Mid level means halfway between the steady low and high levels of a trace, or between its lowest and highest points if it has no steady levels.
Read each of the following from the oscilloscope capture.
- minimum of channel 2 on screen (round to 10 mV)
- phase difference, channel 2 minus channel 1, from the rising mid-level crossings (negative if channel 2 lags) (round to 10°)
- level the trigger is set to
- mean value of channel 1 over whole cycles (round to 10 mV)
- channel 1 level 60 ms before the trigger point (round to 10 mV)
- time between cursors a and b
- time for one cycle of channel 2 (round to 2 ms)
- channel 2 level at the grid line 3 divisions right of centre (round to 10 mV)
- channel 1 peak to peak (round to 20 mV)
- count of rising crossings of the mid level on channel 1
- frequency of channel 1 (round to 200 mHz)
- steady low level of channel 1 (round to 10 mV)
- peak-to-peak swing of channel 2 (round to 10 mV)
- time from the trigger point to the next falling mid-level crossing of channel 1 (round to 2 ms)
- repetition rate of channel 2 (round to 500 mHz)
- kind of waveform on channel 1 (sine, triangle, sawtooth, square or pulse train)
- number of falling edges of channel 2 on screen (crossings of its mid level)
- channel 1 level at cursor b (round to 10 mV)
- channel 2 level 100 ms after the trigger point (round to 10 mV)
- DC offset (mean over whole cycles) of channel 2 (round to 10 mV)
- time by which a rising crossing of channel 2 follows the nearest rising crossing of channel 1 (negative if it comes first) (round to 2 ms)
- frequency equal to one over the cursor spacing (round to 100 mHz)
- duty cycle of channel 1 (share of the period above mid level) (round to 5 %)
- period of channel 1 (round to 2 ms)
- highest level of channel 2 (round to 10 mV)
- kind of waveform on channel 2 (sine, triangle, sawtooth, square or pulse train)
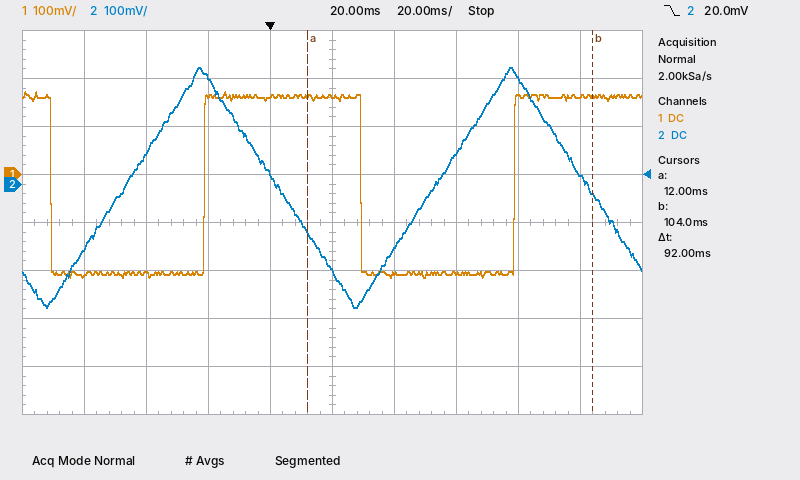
-260 mV
+90°
20.0 mV
-20 mV
-210 mV
92 ms
100 ms
220 mV
380 mV
2
10.0 Hz
-210 mV
500 mV
30 ms
10.0 Hz
square
2
160 mV
20 mV
-10 mV
-26 ms
10.9 Hz
50 %
100 ms
240 mV
triangle
